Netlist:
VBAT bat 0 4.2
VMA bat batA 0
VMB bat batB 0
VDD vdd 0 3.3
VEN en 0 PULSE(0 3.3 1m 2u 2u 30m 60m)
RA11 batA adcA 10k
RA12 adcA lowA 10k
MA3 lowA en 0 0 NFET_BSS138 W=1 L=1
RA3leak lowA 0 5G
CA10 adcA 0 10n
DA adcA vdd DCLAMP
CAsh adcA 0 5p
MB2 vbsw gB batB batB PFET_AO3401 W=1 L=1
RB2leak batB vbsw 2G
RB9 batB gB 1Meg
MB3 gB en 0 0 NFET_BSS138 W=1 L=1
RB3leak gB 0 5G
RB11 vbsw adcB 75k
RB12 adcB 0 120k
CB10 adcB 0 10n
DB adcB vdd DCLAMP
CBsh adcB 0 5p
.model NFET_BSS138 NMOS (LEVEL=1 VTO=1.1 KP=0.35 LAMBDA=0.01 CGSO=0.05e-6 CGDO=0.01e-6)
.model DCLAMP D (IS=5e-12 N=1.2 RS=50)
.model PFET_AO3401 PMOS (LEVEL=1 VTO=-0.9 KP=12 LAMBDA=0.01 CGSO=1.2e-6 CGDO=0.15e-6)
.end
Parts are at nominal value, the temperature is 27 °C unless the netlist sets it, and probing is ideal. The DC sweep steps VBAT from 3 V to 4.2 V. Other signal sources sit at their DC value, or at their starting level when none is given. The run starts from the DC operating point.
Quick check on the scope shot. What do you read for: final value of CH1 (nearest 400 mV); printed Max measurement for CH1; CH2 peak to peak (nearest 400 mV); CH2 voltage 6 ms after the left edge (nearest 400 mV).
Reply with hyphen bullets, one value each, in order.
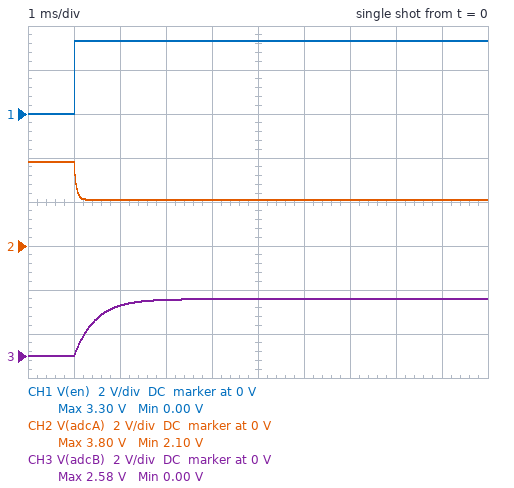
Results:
- 3.2 V
- 3.30 V
- 1.6 V
- 2.0 V
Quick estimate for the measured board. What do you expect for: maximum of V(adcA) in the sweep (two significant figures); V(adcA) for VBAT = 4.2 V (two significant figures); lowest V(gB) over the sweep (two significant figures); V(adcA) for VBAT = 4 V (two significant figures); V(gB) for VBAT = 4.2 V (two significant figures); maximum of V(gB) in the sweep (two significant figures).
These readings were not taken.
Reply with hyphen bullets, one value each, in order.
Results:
- 3.8 V
- 3.8 V
- 3.0 V
- 3.8 V
- 4.2 V
- 4.2 V
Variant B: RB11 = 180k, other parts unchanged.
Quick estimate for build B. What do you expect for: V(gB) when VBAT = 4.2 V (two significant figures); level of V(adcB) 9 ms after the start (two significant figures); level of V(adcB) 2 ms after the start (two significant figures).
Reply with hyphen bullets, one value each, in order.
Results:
- 4.2 V
- 1.7 V
- 1.3 V
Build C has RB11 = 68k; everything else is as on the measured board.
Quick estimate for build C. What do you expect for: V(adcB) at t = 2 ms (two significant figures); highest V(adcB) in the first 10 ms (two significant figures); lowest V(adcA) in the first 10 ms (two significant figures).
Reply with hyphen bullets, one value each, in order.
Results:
- 2.4 V
- 2.7 V
- 2.1 V
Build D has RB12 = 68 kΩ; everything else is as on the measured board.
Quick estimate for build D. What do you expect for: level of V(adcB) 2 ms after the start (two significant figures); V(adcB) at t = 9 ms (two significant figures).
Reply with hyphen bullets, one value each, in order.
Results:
- 1.9 V
- 2.0 V
